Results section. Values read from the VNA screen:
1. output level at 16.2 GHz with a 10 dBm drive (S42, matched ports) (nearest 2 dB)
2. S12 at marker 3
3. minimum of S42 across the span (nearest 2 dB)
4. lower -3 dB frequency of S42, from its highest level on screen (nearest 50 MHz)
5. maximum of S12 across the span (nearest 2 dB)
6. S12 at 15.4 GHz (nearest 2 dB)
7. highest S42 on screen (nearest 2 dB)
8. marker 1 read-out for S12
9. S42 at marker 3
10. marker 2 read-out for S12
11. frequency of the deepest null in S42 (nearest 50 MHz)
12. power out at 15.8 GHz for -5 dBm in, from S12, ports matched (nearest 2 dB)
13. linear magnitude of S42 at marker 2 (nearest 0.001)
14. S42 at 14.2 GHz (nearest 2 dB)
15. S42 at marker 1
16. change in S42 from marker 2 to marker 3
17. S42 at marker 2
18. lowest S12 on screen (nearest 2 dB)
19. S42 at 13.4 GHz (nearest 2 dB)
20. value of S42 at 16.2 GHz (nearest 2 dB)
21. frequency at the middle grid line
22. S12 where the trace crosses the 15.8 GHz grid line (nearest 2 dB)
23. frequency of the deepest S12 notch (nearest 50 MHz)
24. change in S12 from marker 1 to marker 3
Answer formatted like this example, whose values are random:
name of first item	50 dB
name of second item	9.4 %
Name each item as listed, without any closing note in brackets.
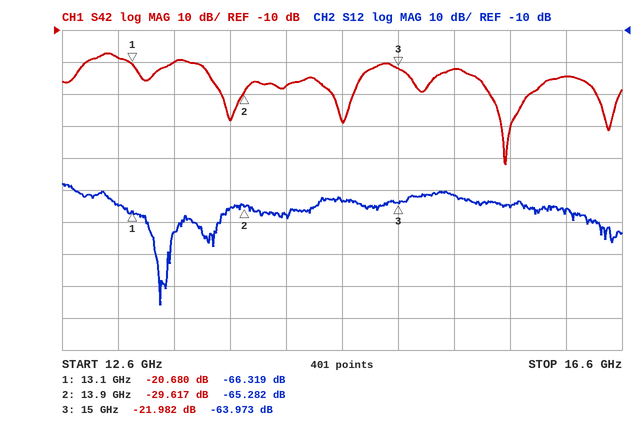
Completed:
output level at 16.2 GHz with a 10 dBm drive (S42, matched ports)	-14 dBm
S12 at marker 3	-63.973 dB
minimum of S42 across the span	-52 dB
lower -3 dB frequency of S42, from its highest level on screen	12.75 GHz
maximum of S12 across the span	-58 dB
S12 at 15.4 GHz	-62 dB
highest S42 on screen	-18 dB
marker 1 read-out for S12	-66.319 dB
S42 at marker 3	-21.982 dB
marker 2 read-out for S12	-65.282 dB
frequency of the deepest null in S42	15.75 GHz
power out at 15.8 GHz for -5 dBm in, from S12, ports matched	-70 dBm
linear magnitude of S42 at marker 2	0.033
S42 at 14.2 GHz	-28 dB
S42 at marker 1	-20.680 dB
change in S42 from marker 2 to marker 3	7.635 dB
S42 at marker 2	-29.617 dB
lowest S12 on screen	-96 dB
S42 at 13.4 GHz	-20 dB
value of S42 at 16.2 GHz	-24 dB
frequency at the middle grid line	14.6 GHz
S12 where the trace crosses the 15.8 GHz grid line	-66 dB
frequency of the deepest S12 notch	13.30 GHz
change in S12 from marker 1 to marker 3	2.346 dB
